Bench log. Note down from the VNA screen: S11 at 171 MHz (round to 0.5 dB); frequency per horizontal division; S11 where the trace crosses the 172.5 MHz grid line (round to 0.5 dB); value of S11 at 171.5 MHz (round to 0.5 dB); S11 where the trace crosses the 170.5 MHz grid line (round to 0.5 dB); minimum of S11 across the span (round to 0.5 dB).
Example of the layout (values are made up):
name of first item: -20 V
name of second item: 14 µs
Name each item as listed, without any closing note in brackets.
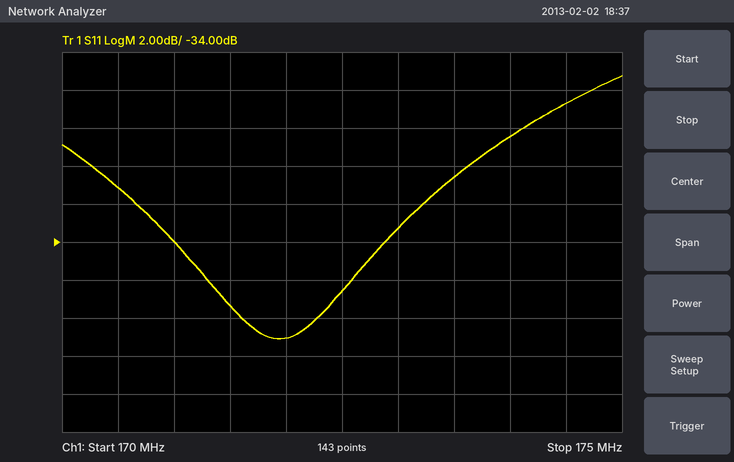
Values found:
S11 at 171 MHz: -34.0 dB
frequency per horizontal division: 500 kHz
S11 where the trace crosses the 172.5 MHz grid line: -36.5 dB
value of S11 at 171.5 MHz: -37.5 dB
S11 where the trace crosses the 170.5 MHz grid line: -31.0 dB
minimum of S11 across the span: -39.0 dB
